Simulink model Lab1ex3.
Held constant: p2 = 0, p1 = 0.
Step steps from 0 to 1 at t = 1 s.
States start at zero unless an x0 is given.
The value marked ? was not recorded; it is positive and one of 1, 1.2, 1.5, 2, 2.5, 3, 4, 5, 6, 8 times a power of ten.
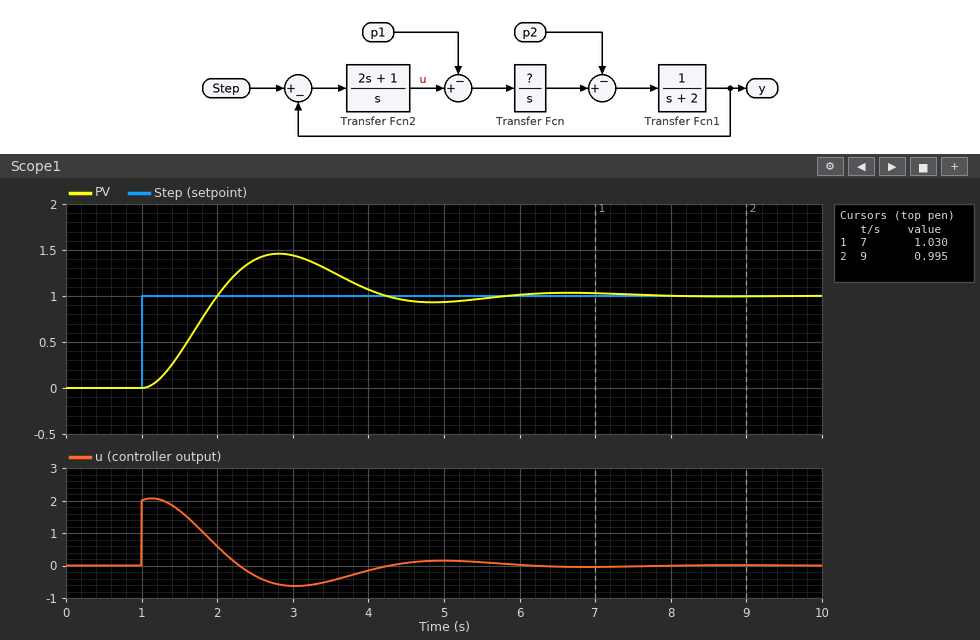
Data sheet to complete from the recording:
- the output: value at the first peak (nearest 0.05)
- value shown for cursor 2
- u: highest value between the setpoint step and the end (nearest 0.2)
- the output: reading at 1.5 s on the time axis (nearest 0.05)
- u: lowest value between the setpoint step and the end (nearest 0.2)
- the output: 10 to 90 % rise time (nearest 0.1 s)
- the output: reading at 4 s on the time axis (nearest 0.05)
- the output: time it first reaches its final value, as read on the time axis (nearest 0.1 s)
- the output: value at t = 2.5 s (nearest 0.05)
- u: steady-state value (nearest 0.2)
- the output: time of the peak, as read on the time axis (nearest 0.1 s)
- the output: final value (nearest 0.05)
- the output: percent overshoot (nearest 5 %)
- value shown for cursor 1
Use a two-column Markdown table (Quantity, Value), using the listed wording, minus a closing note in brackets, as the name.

| Quantity | Value |
|---|---|
| the output: value at the first peak | 1.45 |
| value shown for cursor 2 | 0.995 |
| u: highest value between the setpoint step and the end | 2.0 |
| the output: reading at 1.5 s on the time axis | 0.35 |
| u: lowest value between the setpoint step and the end | -0.6 |
| the output: 10 to 90 % rise time | 0.7 s |
| the output: reading at 4 s on the time axis | 1.05 |
| the output: time it first reaches its final value, as read on the time axis | 2.0 s |
| the output: value at t = 2.5 s | 1.40 |
| u: steady-state value | 0.0 |
| the output: time of the peak, as read on the time axis | 2.8 s |
| the output: final value | 1.00 |
| the output: percent overshoot | 45 % |
| value shown for cursor 1 | 1.030 |
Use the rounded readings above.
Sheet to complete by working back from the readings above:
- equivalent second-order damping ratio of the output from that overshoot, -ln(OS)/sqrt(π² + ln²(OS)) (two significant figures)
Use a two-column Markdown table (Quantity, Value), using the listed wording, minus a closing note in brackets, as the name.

| Quantity | Value |
|---|---|
| equivalent second-order damping ratio of the output from that overshoot, -ln(OS)/sqrt(π² + ln²(OS)) | 0.25 |
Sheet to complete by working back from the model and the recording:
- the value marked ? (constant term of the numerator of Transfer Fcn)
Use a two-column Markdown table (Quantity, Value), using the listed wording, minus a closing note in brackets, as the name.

| Quantity | Value |
|---|---|
| the value marked ? | 2 |
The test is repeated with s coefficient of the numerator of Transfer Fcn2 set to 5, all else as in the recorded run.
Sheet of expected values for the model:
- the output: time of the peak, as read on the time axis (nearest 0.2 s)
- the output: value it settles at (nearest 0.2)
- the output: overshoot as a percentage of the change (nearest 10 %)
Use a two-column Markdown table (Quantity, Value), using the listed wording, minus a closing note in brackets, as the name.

| Quantity | Value |
|---|---|
| the output: time of the peak, as read on the time axis | 2.0 s |
| the output: value it settles at | 1.0 |
| the output: overshoot as a percentage of the change | 40 % |
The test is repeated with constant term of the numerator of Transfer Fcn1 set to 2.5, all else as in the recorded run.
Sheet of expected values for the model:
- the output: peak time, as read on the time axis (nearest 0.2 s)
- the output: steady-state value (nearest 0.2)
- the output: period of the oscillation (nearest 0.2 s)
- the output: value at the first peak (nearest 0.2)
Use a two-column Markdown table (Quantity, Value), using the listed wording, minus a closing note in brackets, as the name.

| Quantity | Value |
|---|---|
| the output: peak time, as read on the time axis | 2.0 s |
| the output: steady-state value | 1.0 |
| the output: period of the oscillation | 2.2 s |
| the output: value at the first peak | 1.6 |
